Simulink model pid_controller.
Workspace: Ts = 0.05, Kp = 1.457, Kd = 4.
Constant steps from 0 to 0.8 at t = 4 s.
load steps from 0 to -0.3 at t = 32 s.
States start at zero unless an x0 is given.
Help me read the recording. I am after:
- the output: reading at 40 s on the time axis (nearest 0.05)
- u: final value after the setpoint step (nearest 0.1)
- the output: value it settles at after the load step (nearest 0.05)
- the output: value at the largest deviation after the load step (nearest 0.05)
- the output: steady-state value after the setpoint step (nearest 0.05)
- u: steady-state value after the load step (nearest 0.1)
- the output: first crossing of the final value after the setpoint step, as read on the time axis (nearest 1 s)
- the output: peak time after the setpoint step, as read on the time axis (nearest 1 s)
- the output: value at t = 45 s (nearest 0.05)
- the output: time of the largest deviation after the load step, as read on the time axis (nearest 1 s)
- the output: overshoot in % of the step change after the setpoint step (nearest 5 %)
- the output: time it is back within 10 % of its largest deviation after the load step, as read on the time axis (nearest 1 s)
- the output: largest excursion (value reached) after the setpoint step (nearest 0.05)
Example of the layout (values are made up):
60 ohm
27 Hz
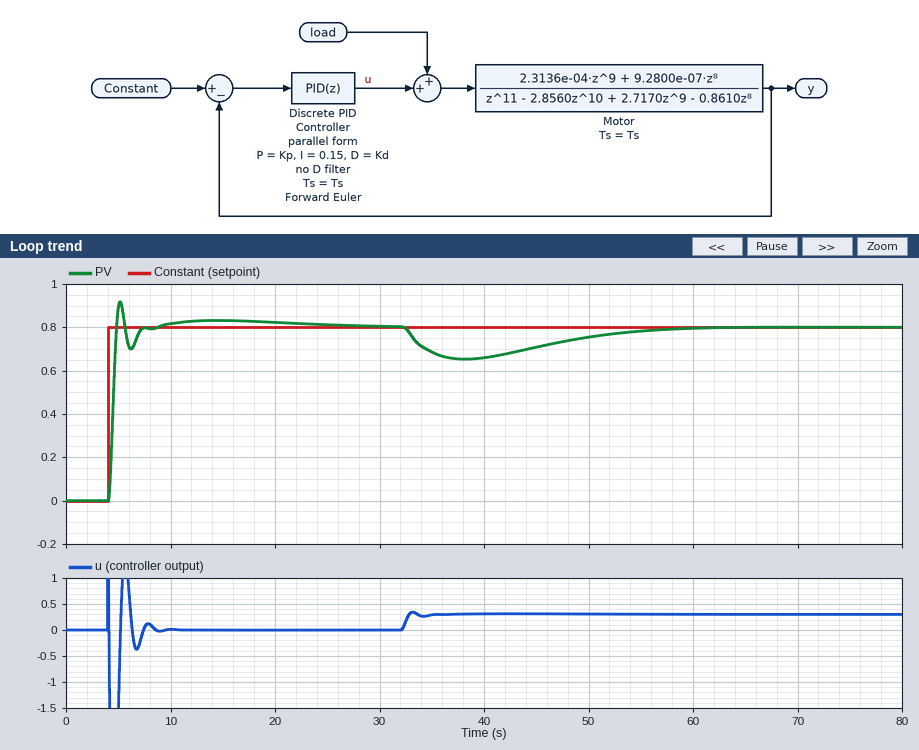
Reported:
0.65
0.0
0.80
0.65
0.80
0.3
5 s
5 s
0.70
38 s
15 %
56 s
0.90
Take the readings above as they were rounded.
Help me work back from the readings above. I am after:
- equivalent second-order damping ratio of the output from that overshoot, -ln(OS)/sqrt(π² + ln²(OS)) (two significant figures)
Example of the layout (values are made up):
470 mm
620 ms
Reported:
0.52
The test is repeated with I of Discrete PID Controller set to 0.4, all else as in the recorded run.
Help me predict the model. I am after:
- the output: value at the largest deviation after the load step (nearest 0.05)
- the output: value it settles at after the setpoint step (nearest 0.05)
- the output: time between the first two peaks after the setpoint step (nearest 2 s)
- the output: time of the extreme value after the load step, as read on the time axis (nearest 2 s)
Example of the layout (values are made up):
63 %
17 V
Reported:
0.70
0.80
6 s
36 s
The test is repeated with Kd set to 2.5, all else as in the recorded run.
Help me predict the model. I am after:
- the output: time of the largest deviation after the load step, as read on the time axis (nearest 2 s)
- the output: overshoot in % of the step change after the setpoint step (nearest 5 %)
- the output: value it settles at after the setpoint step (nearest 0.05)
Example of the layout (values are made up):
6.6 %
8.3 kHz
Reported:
36 s
10 %
0.80
